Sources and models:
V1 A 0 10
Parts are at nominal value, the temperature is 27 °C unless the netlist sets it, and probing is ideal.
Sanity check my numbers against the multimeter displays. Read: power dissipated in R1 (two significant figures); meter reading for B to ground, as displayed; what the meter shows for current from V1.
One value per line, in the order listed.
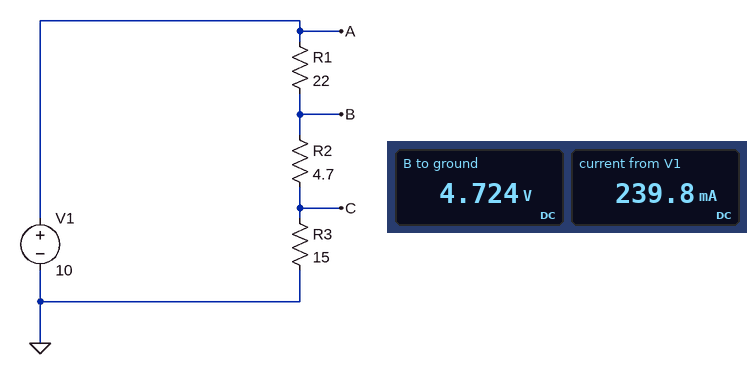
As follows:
1.3 W
4.724 V
239.8 mA
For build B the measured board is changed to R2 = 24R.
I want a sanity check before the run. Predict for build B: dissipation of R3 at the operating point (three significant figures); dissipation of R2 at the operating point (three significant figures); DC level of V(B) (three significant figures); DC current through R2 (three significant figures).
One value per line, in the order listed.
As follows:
403 mW
645 mW
6.39 V
164 mA
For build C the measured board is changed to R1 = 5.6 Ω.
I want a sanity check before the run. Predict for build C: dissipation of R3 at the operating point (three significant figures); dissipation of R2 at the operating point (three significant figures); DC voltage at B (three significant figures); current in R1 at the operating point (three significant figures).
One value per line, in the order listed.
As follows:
2.34 W
734 mW
7.79 V
395 mA
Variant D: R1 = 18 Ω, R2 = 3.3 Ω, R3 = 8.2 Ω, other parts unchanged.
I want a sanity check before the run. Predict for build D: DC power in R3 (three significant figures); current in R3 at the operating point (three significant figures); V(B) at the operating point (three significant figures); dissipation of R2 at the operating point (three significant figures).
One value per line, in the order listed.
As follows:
942 mW
339 mA
3.90 V
379 mW
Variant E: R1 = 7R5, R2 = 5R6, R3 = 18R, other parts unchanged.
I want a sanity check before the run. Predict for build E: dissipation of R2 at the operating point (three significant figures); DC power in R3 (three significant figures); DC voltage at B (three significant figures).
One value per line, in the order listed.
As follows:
579 mW
1.86 W
7.59 V
